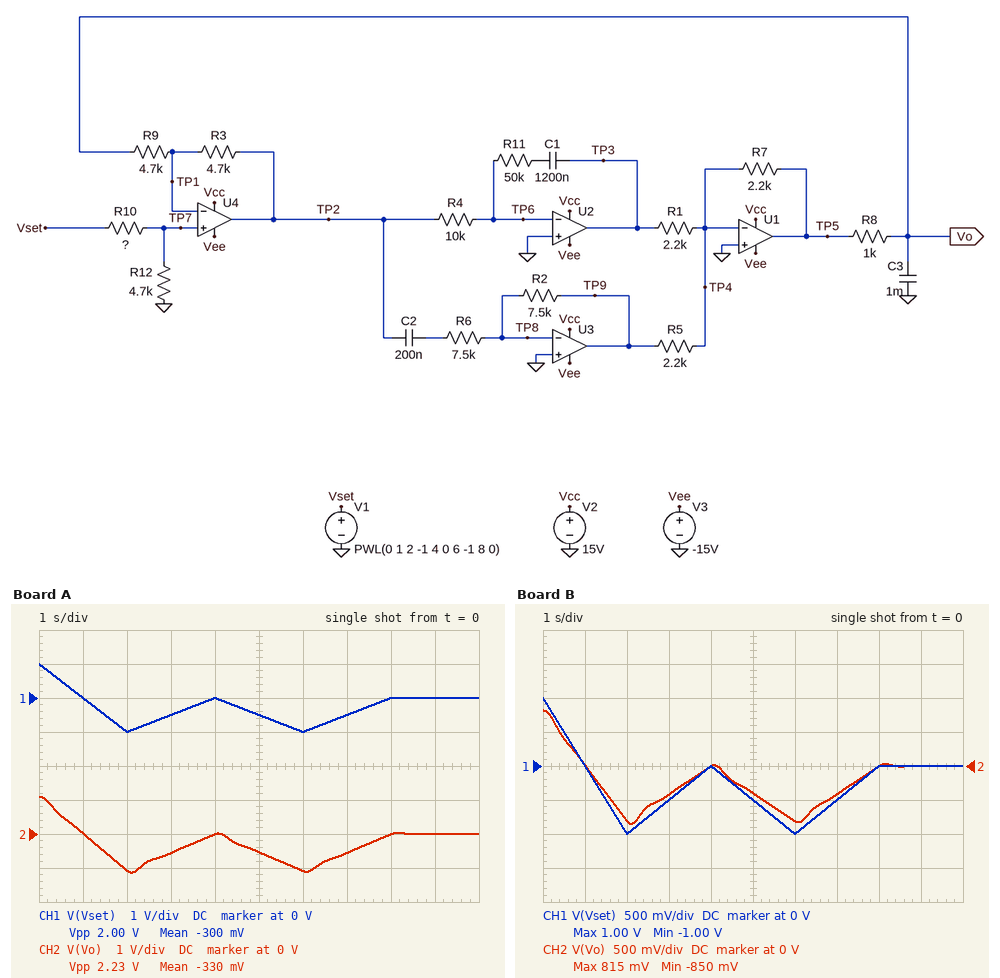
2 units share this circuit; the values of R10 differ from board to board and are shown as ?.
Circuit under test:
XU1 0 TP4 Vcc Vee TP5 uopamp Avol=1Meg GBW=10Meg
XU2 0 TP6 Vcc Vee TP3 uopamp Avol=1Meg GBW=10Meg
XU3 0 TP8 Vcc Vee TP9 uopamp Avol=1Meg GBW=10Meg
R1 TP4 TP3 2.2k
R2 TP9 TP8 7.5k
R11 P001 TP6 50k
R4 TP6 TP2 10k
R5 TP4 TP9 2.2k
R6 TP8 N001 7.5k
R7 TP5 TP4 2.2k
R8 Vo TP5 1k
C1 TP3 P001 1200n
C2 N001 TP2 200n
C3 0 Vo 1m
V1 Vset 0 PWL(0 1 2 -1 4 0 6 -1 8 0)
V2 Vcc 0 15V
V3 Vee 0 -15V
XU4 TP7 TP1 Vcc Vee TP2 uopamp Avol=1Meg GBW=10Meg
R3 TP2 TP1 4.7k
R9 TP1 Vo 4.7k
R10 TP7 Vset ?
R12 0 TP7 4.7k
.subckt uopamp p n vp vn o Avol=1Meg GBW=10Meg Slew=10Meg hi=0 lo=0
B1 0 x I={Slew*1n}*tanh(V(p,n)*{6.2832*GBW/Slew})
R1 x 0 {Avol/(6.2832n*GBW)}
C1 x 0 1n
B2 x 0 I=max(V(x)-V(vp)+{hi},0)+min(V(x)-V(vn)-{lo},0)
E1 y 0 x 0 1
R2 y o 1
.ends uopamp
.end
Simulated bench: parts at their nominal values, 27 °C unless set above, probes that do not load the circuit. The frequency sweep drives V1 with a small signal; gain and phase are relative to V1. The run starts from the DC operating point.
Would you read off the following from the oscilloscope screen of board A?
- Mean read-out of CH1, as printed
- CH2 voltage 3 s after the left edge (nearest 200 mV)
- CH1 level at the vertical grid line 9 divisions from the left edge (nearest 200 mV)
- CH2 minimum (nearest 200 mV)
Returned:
-300 mV
-600 mV
0 V
-1.2 V
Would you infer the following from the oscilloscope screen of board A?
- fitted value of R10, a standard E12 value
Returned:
3.9 kΩ
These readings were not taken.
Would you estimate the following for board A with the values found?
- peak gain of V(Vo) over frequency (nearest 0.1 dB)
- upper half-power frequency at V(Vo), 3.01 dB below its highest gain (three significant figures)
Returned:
5.6 dB
1.79 Hz
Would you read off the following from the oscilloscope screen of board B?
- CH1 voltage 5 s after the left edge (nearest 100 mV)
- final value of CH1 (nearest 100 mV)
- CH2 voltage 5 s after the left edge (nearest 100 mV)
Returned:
-500 mV
0 V
-400 mV
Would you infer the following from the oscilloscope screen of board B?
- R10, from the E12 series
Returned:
6.8 kΩ
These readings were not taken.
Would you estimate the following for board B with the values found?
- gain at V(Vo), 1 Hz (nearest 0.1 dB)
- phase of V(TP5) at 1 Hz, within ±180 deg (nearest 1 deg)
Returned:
1.9 dB
59 deg
